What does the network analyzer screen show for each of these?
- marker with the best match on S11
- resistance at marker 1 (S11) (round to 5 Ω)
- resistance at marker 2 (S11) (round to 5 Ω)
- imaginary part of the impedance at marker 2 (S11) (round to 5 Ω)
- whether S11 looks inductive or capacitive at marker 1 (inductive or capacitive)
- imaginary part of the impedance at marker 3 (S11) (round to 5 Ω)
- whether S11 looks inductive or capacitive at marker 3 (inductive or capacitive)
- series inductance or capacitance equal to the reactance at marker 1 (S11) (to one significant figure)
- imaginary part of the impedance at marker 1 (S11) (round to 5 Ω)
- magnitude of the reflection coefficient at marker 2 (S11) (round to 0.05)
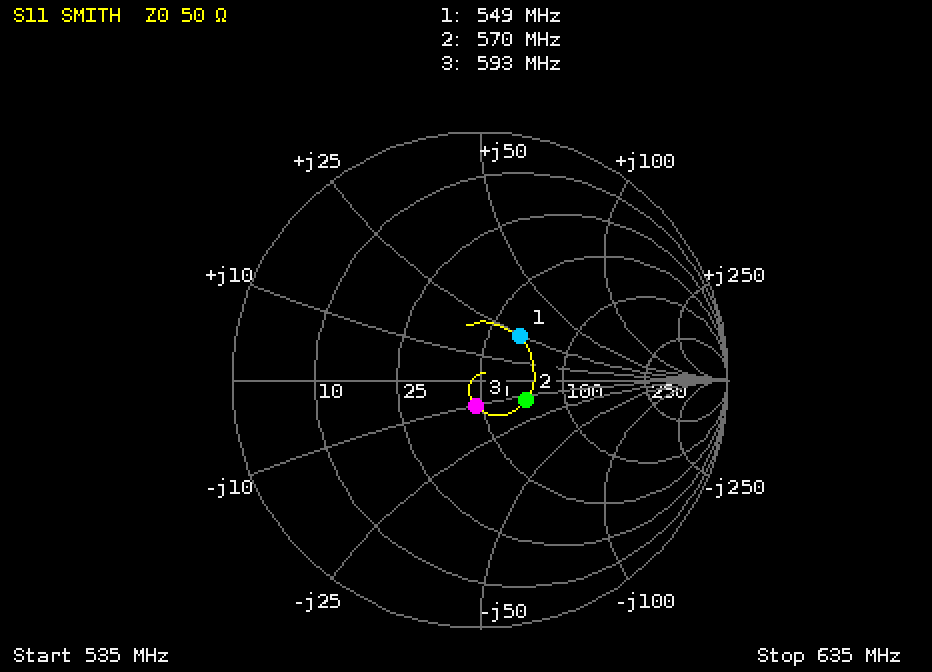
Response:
marker 3
65 Ω
70 Ω
-10 Ω
inductive
-10 Ω
capacitive
7 nH
+25 Ω
0.20
